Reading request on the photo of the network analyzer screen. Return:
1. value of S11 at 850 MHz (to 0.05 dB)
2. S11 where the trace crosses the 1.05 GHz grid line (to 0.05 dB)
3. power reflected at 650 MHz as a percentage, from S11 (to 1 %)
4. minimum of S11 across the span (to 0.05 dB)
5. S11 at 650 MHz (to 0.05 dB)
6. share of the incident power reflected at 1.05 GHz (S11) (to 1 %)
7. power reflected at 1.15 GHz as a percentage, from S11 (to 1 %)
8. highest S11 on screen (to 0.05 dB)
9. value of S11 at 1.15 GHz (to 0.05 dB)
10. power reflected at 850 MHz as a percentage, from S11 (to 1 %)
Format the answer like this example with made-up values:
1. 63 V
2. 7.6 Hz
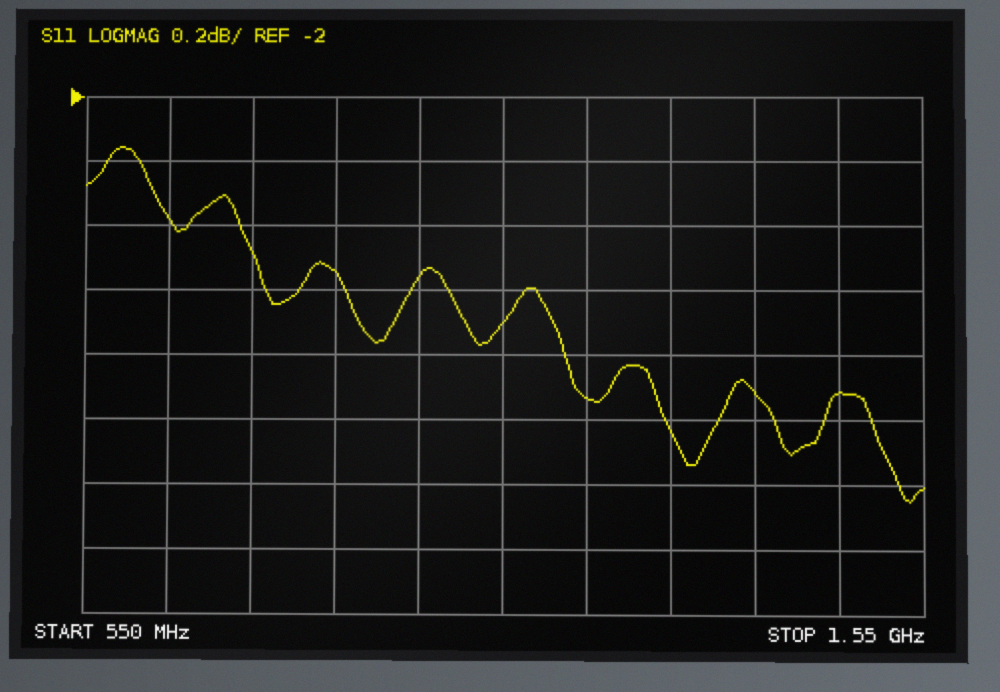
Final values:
1. -2.55 dB
2. -2.70 dB
3. 58 %
4. -3.25 dB
5. -2.40 dB
6. 54 %
7. 51 %
8. -2.15 dB
9. -2.95 dB
10. 56 %
